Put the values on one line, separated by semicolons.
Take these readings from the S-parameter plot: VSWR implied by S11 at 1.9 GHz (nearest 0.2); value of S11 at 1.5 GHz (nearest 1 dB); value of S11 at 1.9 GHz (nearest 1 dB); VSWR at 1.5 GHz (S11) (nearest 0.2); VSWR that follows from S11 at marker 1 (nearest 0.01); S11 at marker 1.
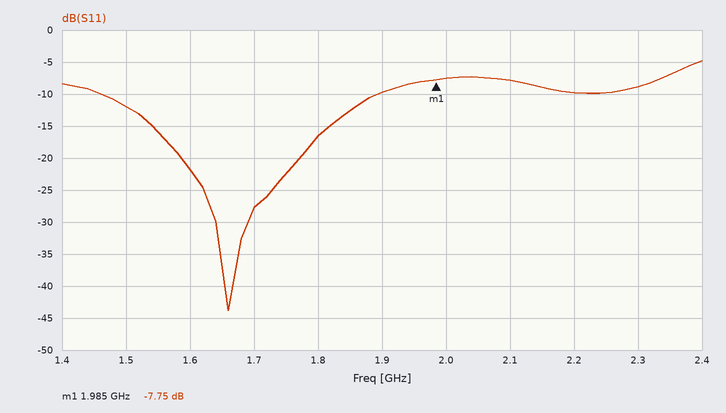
2.0; -12 dB; -10 dB; 1.6; 2.39; -7.75 dB
